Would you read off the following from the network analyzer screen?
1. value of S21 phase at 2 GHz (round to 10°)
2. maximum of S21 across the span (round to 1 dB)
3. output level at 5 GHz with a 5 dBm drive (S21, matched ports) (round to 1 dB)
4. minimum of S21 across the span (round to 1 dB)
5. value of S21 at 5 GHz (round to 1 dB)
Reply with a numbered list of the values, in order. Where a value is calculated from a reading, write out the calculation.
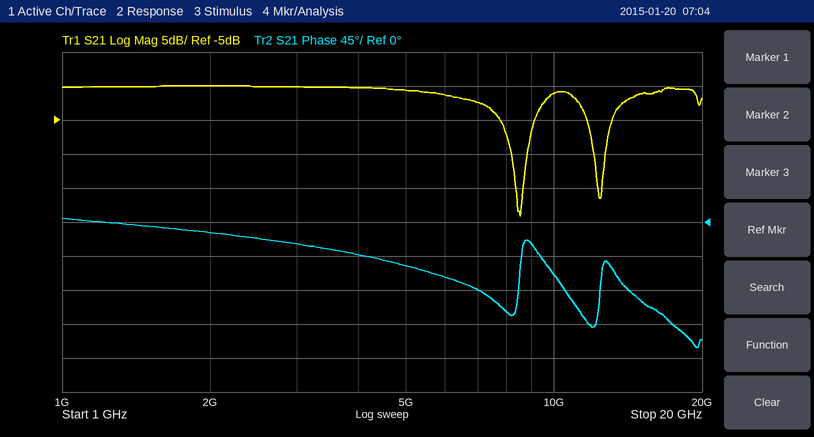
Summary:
1. -10°
2. 0 dB
3. 5 dBm + (-1 dB) = 4 dBm
4. -19 dB
5. -1 dB
